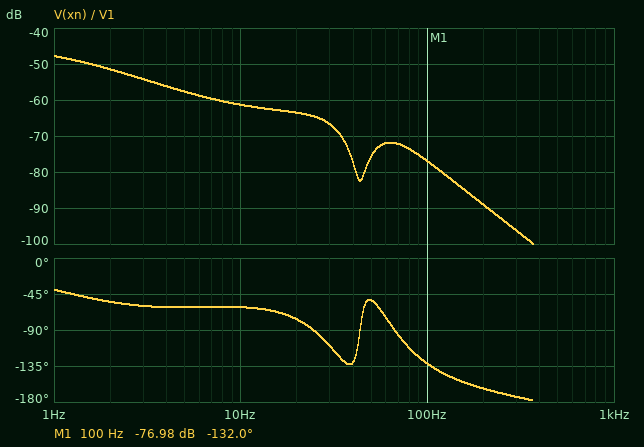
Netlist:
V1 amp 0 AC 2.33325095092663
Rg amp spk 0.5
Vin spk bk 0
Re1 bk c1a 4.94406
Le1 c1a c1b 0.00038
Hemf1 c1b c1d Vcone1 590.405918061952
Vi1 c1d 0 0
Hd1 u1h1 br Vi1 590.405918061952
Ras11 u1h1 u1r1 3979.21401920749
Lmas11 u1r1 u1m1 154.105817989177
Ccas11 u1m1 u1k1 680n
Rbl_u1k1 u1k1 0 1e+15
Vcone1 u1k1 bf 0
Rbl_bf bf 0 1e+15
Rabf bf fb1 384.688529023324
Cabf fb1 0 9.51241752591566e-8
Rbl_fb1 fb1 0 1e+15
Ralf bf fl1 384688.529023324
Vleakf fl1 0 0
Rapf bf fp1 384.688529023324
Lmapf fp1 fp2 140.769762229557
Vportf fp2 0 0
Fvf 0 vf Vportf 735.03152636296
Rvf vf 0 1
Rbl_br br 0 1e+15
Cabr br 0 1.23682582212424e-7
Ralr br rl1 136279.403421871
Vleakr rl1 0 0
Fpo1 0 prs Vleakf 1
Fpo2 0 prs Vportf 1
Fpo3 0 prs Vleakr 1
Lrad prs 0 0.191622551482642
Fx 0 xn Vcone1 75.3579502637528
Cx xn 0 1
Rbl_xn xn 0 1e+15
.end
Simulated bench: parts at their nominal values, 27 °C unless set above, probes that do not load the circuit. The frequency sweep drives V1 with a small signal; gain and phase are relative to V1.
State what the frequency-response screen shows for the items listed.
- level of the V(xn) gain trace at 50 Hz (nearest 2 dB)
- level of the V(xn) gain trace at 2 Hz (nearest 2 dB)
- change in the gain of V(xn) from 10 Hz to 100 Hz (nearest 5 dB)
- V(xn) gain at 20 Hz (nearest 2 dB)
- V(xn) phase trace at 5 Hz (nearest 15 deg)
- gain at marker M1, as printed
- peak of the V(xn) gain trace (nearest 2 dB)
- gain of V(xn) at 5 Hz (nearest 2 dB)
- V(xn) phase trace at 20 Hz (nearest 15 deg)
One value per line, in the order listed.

-76 dB
-52 dB
-15 dB
-64 dB
-60 deg
-76.98 dB
-48 dB
-58 dB
-75 deg
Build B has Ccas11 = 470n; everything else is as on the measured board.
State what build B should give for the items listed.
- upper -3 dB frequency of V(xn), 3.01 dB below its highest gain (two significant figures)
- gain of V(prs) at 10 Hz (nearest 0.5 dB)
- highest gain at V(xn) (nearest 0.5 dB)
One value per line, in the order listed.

1.5 Hz
-44.0 dB
-48.5 dB
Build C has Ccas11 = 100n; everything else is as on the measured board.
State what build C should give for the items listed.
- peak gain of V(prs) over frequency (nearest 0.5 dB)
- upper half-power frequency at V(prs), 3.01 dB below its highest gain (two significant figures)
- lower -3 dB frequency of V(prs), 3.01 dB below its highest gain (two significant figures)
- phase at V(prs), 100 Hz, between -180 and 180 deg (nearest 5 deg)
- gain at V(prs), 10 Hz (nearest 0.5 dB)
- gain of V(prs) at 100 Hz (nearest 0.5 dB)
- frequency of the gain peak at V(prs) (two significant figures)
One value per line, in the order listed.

-18.0 dB
62 Hz
31 Hz
-130 deg
-48.0 dB
-28.5 dB
39 Hz
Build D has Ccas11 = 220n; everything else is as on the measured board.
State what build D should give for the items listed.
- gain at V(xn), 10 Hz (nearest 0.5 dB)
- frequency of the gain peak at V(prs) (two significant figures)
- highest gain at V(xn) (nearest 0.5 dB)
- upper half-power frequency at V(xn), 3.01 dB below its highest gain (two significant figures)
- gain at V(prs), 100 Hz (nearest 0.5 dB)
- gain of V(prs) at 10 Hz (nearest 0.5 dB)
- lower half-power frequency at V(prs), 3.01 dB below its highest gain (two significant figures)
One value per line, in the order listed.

-63.0 dB
43 Hz
-55.0 dB
3.1 Hz
-29.0 dB
-45.0 dB
31 Hz
